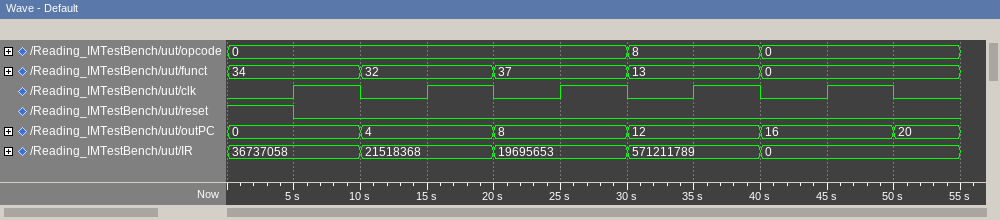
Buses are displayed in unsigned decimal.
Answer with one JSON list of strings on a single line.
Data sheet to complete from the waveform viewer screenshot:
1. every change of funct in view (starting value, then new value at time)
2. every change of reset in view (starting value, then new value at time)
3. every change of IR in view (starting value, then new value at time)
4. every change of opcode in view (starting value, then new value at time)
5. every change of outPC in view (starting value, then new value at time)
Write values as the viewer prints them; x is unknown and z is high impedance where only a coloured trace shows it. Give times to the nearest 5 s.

["34, 32 at 10 s, 37 at 20 s, 13 at 30 s, 0 at 40 s", "1, 0 at 5 s", "36737058, 21518368 at 10 s, 19695653 at 20 s, 571211789 at 30 s, 0 at 40 s", "0, 8 at 30 s, 0 at 40 s", "0, 4 at 10 s, 8 at 20 s, 12 at 30 s, 16 at 40 s, 20 at 50 s"]
